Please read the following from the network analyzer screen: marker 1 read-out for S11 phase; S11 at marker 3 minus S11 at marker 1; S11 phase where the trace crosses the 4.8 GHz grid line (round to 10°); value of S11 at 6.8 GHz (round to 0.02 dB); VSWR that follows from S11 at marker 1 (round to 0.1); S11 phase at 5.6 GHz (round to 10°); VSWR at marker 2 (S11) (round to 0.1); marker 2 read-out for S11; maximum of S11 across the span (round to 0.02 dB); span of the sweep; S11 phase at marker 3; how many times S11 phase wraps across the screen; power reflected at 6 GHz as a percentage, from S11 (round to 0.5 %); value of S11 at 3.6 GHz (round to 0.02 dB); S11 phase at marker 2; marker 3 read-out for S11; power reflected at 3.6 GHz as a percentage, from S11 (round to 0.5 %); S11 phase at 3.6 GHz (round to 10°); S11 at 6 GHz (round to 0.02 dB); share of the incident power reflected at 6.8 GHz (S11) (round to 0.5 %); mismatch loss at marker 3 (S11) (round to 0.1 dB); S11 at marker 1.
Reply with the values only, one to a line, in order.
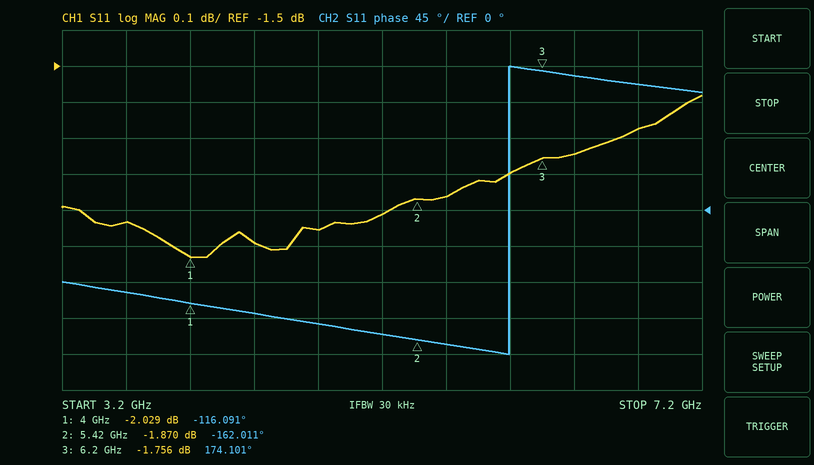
-116.091°
0.273 dB
-140°
-1.68 dB
8.6
-170°
9.3
-1.870 dB
-1.58 dB
4 GHz
174.101°
1
66.0 %
-1.94 dB
-162.011°
-1.756 dB
64.0 %
-100°
-1.80 dB
68.0 %
4.8 dB
-2.029 dB
